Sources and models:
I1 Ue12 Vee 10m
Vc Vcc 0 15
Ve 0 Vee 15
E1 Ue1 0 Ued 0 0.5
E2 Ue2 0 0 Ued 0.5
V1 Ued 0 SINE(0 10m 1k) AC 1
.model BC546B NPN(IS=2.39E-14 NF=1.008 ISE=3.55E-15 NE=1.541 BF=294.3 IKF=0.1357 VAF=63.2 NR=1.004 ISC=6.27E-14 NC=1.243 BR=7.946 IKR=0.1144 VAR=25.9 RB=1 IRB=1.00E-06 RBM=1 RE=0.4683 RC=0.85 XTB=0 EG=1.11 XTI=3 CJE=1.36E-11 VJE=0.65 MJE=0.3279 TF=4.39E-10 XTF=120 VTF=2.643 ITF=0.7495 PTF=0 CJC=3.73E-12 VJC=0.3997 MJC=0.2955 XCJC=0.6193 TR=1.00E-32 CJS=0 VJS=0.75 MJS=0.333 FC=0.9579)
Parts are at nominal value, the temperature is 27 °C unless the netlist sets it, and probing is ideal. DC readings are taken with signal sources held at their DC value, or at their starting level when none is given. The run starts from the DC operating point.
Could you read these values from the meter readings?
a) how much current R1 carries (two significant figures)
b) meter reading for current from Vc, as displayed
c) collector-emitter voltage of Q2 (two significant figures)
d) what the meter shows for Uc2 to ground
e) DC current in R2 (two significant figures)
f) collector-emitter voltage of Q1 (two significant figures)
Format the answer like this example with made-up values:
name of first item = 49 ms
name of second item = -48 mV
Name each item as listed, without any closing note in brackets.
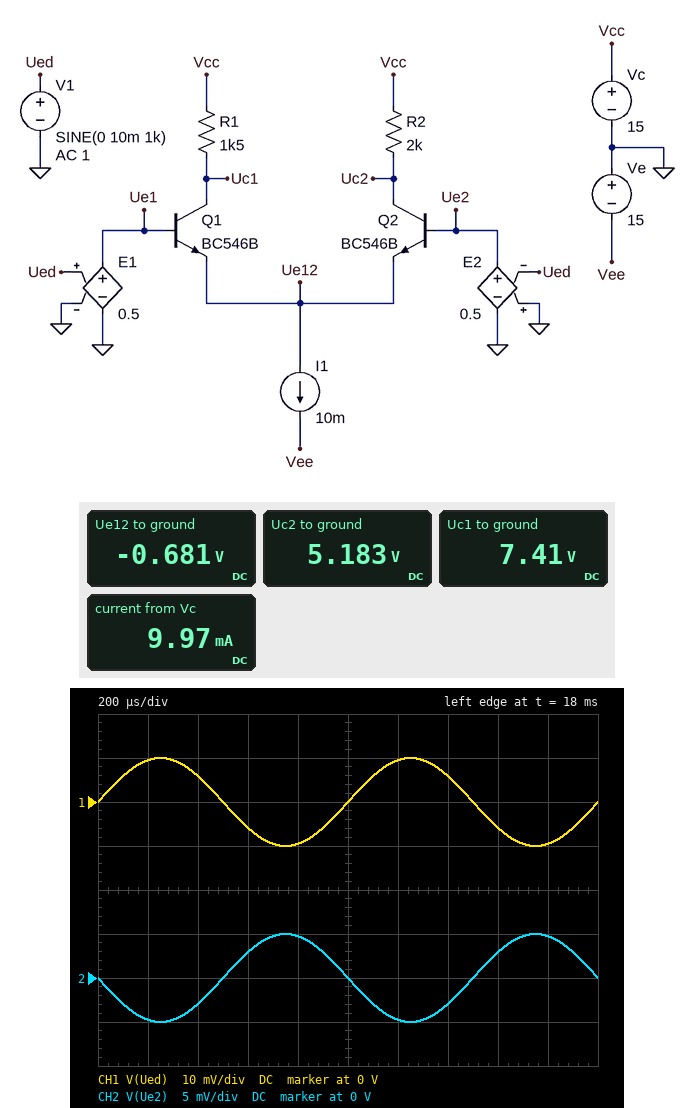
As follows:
how much current R1 carries = 5.1 mA
meter reading for current from Vc, as displayed = 9.97 mA
collector-emitter voltage of Q2 = 5.9 V
what the meter shows for Uc2 to ground = 5.183 V
DC current in R2 = 4.9 mA
collector-emitter voltage of Q1 = 8.1 V
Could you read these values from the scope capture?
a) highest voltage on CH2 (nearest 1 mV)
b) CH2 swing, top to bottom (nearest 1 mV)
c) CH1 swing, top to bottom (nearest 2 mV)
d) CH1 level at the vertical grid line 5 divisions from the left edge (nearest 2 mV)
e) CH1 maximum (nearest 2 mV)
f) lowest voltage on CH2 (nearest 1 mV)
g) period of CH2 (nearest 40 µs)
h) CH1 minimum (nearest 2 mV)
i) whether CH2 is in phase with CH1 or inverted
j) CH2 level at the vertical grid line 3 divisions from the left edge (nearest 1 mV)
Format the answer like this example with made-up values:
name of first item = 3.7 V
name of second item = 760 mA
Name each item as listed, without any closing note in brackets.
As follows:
highest voltage on CH2 = 5 mV
CH2 swing, top to bottom = 10 mV
CH1 swing, top to bottom = 20 mV
CH1 level at the vertical grid line 5 divisions from the left edge = 0 V
CH1 maximum = 10 mV
lowest voltage on CH2 = -5 mV
period of CH2 = 1.00 ms
CH1 minimum = -10 mV
whether CH2 is in phase with CH1 or inverted = inverted
CH2 level at the vertical grid line 3 divisions from the left edge = 3 mV
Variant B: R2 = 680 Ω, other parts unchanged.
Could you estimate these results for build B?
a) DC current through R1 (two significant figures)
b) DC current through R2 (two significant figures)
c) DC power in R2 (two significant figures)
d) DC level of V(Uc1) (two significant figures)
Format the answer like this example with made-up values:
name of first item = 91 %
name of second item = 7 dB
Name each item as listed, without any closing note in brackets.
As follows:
DC current through R1 = 4.9 mA
DC current through R2 = 5.1 mA
DC power in R2 = 18 mW
DC level of V(Uc1) = 7.7 V
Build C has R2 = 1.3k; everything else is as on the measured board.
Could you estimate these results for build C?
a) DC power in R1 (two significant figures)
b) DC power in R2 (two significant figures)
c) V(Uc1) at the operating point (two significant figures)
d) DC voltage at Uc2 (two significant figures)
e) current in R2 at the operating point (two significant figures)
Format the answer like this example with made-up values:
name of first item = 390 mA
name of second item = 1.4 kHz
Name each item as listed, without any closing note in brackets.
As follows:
DC power in R1 = 37 mW
DC power in R2 = 33 mW
V(Uc1) at the operating point = 7.6 V
DC voltage at Uc2 = 8.5 V
current in R2 at the operating point = 5.0 mA
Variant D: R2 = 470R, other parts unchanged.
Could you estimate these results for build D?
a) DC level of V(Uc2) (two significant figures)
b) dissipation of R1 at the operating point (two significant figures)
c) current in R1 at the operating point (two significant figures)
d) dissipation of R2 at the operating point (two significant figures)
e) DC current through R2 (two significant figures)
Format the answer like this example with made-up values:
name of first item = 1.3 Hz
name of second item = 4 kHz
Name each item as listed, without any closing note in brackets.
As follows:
DC level of V(Uc2) = 13 V
dissipation of R1 at the operating point = 35 mW
current in R1 at the operating point = 4.8 mA
dissipation of R2 at the operating point = 12 mW
DC current through R2 = 5.1 mA
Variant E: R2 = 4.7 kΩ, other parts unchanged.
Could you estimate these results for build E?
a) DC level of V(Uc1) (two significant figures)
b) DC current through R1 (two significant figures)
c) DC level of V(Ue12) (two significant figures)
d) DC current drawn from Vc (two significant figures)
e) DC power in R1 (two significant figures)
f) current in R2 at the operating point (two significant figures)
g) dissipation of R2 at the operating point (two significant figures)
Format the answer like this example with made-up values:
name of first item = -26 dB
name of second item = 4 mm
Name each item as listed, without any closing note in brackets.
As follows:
DC level of V(Uc1) = 5.6 V
DC current through R1 = 6.3 mA
DC level of V(Ue12) = -690 mV
DC current drawn from Vc = 9.6 mA
DC power in R1 = 59 mW
current in R2 at the operating point = 3.3 mA
dissipation of R2 at the operating point = 52 mW
